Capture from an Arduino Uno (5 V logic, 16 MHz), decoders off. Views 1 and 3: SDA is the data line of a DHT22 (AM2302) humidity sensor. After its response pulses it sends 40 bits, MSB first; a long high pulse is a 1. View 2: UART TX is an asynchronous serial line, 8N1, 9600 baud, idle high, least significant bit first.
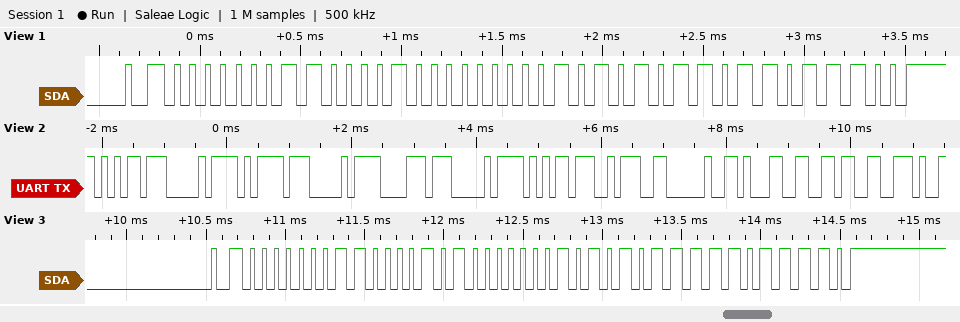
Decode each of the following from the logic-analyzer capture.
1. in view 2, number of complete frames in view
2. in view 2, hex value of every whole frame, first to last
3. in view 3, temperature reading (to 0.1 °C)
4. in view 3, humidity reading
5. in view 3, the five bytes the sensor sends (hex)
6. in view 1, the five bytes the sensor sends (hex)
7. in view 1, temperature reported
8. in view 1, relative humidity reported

12
0xB5 0xD0 0xBD 0xD0 0xB8 0xD0 0xB5 0x3A 0x20 0x31 0x36 0x2E
34.3 °C
38.9 %
01 85 01 57 DE
01 84 01 56 DC
34.2 °C
38.8 %
